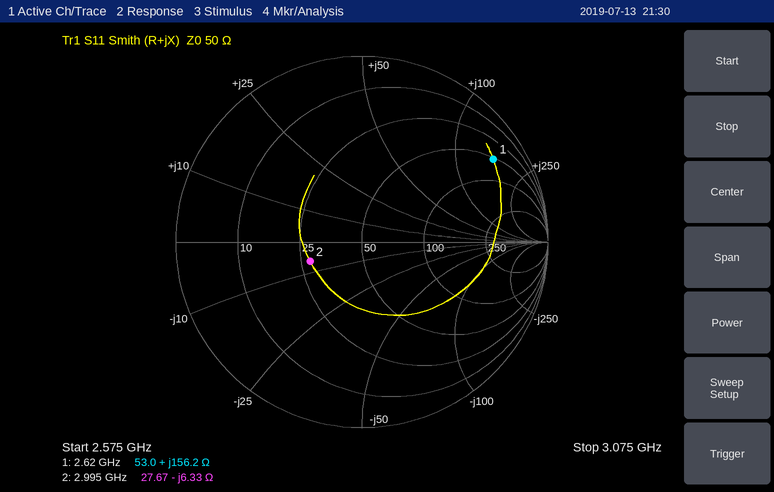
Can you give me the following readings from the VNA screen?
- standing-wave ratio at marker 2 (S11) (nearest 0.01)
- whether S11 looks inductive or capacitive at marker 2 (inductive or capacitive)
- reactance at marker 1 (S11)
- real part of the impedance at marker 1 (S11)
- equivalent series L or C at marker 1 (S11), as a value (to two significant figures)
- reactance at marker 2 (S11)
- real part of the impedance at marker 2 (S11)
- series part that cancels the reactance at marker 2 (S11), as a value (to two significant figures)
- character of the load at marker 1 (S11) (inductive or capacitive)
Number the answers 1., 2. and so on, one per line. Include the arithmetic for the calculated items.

1. 1.85
2. capacitive
3. +156.2 Ω
4. 53.0 Ω
5. L = 156.2 Ω/(2π × 2.62 GHz) ≈ 9.5 nH
6. -6.33 Ω
7. 27.67 Ω
8. L = 6.33 Ω/(2π × 2.995 GHz) ≈ 336 pH, so 340 pH to two significant figures
9. inductive
